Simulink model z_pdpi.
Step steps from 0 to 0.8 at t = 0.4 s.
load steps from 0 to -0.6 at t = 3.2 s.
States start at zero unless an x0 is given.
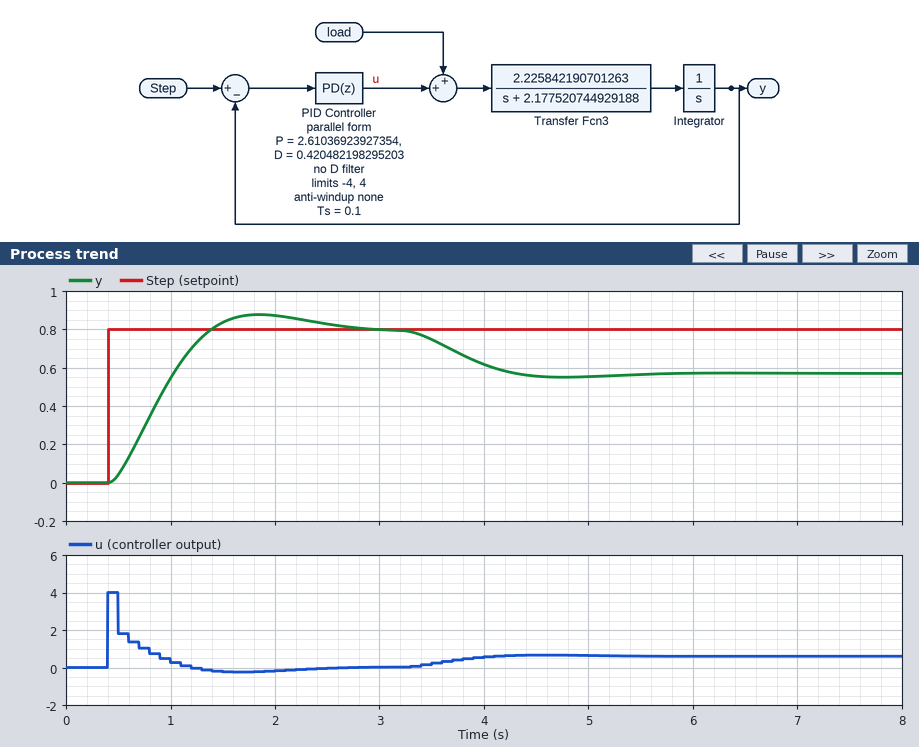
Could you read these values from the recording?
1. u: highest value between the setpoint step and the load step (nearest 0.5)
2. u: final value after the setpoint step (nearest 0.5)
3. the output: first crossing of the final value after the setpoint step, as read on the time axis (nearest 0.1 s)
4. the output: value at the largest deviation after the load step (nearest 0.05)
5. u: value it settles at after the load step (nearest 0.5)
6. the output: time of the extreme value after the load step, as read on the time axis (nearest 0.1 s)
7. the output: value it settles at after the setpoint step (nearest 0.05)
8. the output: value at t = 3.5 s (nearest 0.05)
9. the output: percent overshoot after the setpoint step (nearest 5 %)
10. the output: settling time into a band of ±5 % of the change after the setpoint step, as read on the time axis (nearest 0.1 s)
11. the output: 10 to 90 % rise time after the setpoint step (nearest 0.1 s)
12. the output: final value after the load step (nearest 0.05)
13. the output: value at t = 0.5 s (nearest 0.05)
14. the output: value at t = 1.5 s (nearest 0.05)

4.0
0.0
1.4 s
0.55
0.5
4.8 s
0.80
0.75
10 %
2.4 s
0.7 s
0.55
0.05
0.85
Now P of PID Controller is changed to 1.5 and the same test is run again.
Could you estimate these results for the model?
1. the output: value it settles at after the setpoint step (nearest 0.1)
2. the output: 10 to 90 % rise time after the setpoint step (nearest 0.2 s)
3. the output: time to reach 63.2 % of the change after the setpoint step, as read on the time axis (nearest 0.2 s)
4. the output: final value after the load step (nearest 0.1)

0.8
1.2 s
1.2 s
0.4
